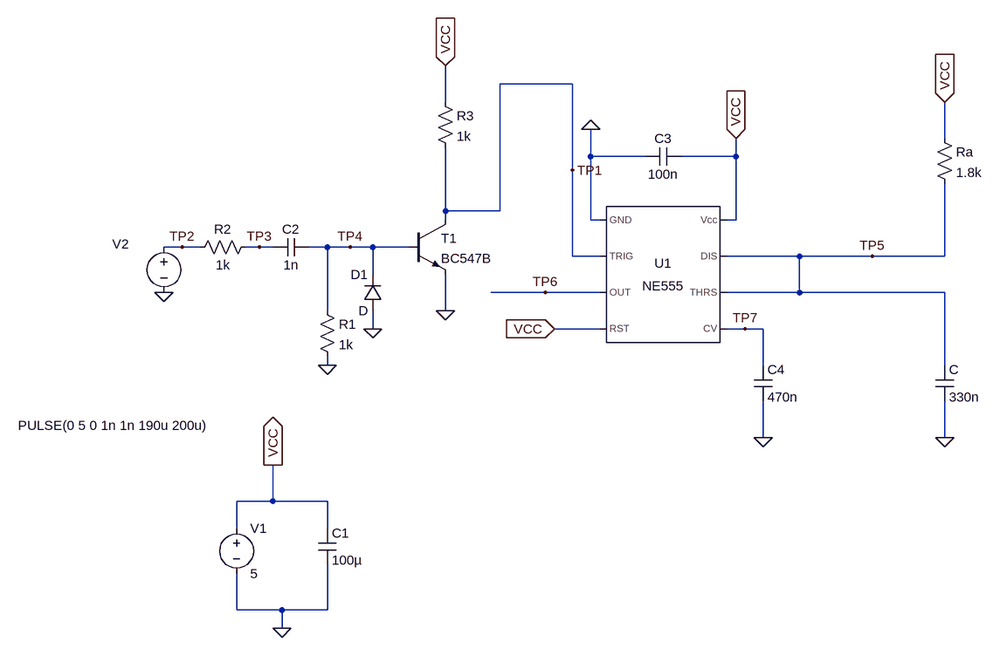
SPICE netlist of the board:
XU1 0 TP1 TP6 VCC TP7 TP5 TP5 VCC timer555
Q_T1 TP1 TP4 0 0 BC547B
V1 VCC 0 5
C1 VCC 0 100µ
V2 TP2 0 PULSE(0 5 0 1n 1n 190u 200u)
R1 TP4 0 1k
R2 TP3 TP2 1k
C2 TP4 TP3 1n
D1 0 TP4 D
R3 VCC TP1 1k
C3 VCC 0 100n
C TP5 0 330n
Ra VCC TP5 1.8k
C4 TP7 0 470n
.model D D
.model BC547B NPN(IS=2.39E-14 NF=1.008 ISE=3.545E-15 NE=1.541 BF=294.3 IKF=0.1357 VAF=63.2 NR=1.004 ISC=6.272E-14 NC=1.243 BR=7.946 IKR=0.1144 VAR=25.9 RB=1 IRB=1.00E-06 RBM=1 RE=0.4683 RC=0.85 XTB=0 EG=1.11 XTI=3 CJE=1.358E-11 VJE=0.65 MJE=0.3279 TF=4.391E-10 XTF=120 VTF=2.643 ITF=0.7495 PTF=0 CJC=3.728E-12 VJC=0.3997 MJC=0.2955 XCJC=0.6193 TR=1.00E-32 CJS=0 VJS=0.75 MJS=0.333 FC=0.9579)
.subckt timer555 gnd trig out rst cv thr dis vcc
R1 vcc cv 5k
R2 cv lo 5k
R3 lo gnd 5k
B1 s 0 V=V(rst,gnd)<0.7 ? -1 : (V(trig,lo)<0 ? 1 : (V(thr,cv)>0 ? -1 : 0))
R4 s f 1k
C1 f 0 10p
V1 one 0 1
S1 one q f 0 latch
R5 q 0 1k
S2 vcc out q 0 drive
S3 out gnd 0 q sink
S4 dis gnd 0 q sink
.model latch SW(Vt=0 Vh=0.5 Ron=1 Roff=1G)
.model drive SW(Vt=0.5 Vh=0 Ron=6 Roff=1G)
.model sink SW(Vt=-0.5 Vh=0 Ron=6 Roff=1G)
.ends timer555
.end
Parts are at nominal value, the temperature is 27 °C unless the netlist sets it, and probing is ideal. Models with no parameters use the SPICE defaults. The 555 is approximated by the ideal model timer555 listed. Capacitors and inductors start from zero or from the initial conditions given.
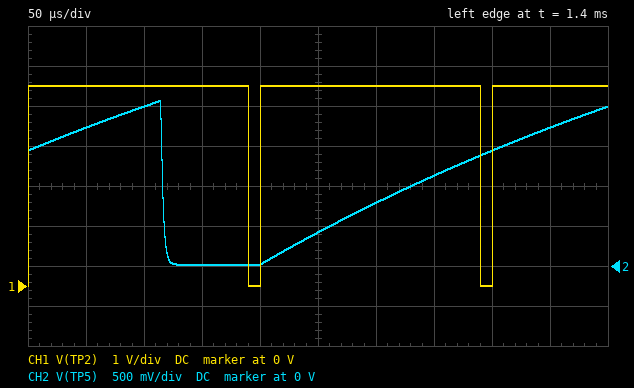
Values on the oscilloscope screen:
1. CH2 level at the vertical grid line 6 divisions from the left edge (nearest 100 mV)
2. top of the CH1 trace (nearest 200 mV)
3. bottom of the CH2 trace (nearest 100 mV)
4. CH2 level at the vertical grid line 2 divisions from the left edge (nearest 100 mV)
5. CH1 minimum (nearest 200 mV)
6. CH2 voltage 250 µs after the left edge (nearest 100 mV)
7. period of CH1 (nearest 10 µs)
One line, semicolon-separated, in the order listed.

800 mV; 5.0 V; 0 V; 2.0 V; 0 V; 400 mV; 200 µs
